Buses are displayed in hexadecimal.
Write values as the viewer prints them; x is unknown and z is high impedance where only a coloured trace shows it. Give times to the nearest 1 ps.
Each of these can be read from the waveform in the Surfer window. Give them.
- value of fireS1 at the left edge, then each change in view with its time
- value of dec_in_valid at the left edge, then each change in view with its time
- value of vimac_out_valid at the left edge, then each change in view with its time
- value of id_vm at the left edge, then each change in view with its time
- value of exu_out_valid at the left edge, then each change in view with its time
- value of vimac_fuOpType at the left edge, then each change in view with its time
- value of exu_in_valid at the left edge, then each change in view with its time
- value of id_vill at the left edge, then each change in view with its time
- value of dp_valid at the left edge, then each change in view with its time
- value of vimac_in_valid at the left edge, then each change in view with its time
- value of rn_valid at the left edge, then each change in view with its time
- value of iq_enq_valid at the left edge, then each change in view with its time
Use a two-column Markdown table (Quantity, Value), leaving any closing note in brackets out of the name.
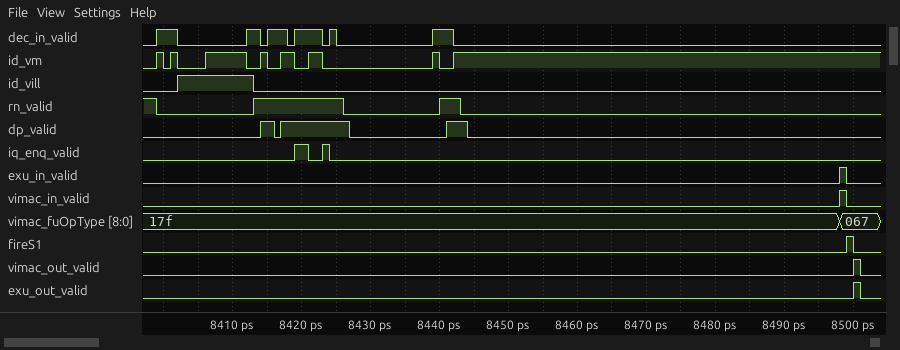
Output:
| Quantity | Value |
|---|---|
| value of fireS1 at the left edge, then each change in view with its time | 0, 1 at 8499 ps, 0 at 8500 ps |
| value of dec_in_valid at the left edge, then each change in view with its time | 0, 1 at 8399 ps, 0 at 8402 ps, 1 at 8412 ps, 0 at 8414 ps, 1 at 8415 ps, 0 at 8418 ps, 1 at 8419 ps, 0 at 8423 ps, 1 at 8424 ps, 0 at 8425 ps, 1 at 8439 ps, 0 at 8442 ps |
| value of vimac_out_valid at the left edge, then each change in view with its time | 0, 1 at 8500 ps, 0 at 8501 ps |
| value of id_vm at the left edge, then each change in view with its time | 0, 1 at 8399 ps, 0 at 8400 ps, 1 at 8401 ps, 0 at 8402 ps, 1 at 8406 ps, 0 at 8412 ps, 1 at 8414 ps, 0 at 8415 ps, 1 at 8417 ps, 0 at 8419 ps, 1 at 8421 ps, 0 at 8423 ps, 1 at 8439 ps, 0 at 8440 ps, 1 at 8442 ps |
| value of exu_out_valid at the left edge, then each change in view with its time | 0, 1 at 8500 ps, 0 at 8501 ps |
| value of vimac_fuOpType at the left edge, then each change in view with its time | 17f, 067 at 8498 ps |
| value of exu_in_valid at the left edge, then each change in view with its time | 0, 1 at 8498 ps, 0 at 8499 ps |
| value of id_vill at the left edge, then each change in view with its time | 0, 1 at 8402 ps, 0 at 8413 ps |
| value of dp_valid at the left edge, then each change in view with its time | 0, 1 at 8414 ps, 0 at 8416 ps, 1 at 8417 ps, 0 at 8427 ps, 1 at 8441 ps, 0 at 8444 ps |
| value of vimac_in_valid at the left edge, then each change in view with its time | 0, 1 at 8498 ps, 0 at 8499 ps |
| value of rn_valid at the left edge, then each change in view with its time | 1, 0 at 8399 ps, 1 at 8413 ps, 0 at 8426 ps, 1 at 8440 ps, 0 at 8443 ps |
| value of iq_enq_valid at the left edge, then each change in view with its time | 0, 1 at 8419 ps, 0 at 8421 ps, 1 at 8423 ps, 0 at 8424 ps |
